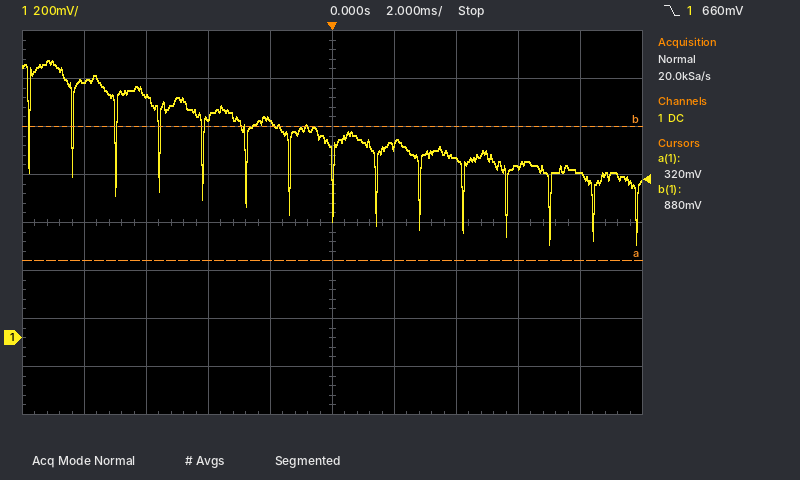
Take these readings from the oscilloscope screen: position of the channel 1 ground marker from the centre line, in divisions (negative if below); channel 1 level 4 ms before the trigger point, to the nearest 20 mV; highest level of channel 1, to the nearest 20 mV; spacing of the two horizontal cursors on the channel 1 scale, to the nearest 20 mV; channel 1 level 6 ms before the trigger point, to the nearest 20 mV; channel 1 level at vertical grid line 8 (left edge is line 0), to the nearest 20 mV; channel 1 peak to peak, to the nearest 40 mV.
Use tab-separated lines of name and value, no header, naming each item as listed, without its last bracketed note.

position of the channel 1 ground marker from the centre line, in divisions	-2.4 div
channel 1 level 4 ms before the trigger point, to the nearest 20 mV	920 mV
highest level of channel 1, to the nearest 20 mV	1.16 V
spacing of the two horizontal cursors on the channel 1 scale, to the nearest 20 mV	560 mV
channel 1 level 6 ms before the trigger point, to the nearest 20 mV	1.00 V
channel 1 level at vertical grid line 8 (left edge is line 0), to the nearest 20 mV	720 mV
channel 1 peak to peak, to the nearest 40 mV	760 mV
